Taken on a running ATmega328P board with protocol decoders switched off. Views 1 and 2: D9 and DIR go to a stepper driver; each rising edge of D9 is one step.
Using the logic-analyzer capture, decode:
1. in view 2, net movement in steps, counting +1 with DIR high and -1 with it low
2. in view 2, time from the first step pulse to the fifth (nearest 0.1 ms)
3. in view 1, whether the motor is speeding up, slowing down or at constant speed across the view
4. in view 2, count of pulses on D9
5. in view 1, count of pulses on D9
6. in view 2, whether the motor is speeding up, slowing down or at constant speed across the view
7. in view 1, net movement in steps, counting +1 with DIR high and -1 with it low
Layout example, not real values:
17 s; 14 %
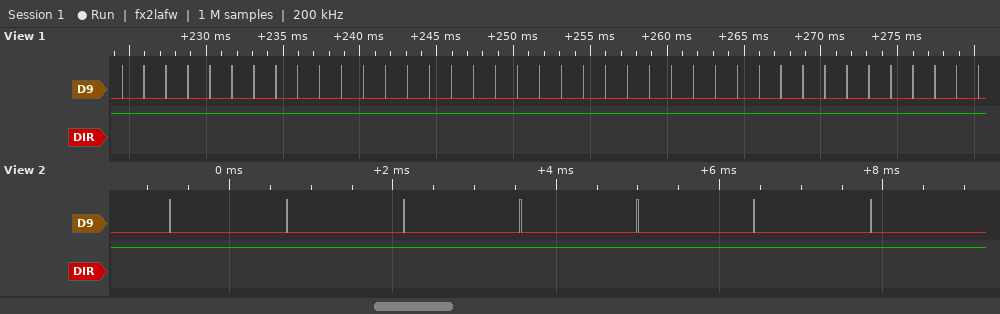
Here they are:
+7; 5.7 ms; constant speed; 7; 40; constant speed; +40
